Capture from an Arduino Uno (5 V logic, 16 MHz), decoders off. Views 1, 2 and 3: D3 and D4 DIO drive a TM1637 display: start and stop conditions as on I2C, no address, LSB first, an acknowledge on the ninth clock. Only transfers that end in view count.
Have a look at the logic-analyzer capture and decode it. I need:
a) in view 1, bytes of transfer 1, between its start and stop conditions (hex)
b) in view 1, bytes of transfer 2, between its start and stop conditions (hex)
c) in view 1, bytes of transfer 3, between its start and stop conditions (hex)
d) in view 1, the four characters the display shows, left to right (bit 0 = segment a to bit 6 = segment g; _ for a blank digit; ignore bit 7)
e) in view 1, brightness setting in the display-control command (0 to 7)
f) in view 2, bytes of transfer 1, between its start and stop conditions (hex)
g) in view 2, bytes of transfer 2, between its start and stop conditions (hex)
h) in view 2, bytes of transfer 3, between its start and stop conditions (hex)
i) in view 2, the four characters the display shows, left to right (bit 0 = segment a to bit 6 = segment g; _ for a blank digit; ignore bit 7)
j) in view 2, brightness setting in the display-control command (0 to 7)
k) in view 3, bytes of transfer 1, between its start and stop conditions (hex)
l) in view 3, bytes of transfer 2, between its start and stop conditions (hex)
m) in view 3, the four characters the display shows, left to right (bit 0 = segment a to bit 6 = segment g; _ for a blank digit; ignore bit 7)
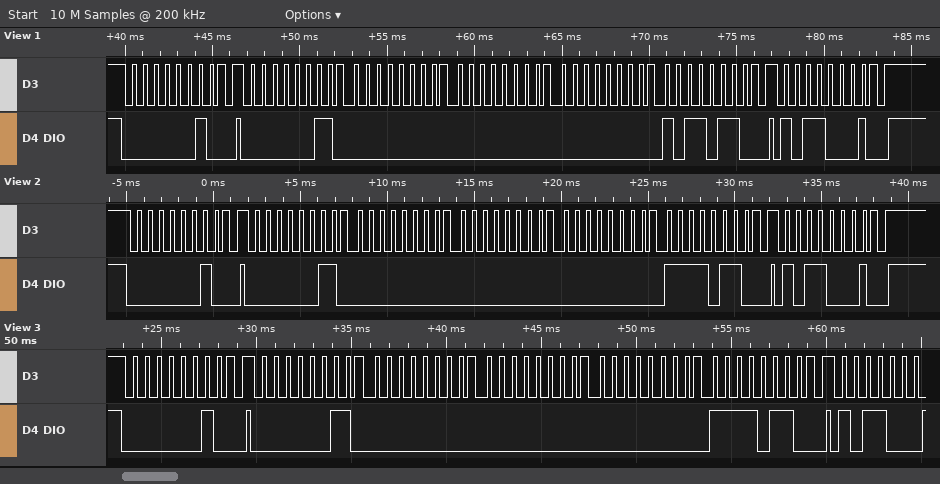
40
C0 00 00 00 6D
8D
___5
5
40
C0 00 00 00 6F
8D
___9
5
40
C0 00 00 00 6F
___9
